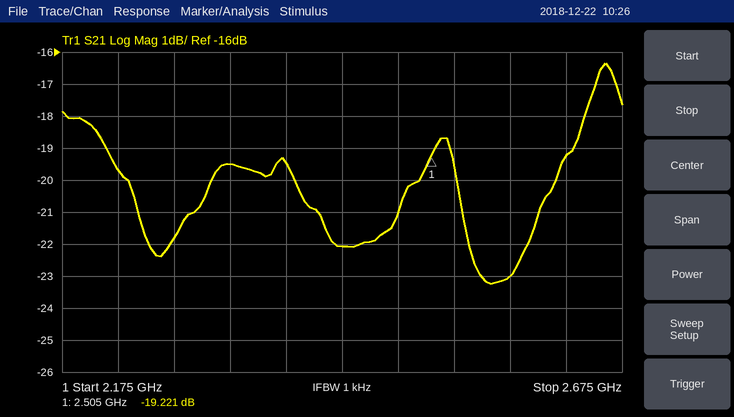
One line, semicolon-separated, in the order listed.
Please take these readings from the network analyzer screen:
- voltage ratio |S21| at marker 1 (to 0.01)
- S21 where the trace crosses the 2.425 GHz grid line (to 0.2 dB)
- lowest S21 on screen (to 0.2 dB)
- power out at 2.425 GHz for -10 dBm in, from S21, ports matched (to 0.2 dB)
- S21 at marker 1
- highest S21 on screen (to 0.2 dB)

0.11; -22.0 dB; -23.2 dB; -32.0 dBm; -19.221 dB; -16.4 dB
